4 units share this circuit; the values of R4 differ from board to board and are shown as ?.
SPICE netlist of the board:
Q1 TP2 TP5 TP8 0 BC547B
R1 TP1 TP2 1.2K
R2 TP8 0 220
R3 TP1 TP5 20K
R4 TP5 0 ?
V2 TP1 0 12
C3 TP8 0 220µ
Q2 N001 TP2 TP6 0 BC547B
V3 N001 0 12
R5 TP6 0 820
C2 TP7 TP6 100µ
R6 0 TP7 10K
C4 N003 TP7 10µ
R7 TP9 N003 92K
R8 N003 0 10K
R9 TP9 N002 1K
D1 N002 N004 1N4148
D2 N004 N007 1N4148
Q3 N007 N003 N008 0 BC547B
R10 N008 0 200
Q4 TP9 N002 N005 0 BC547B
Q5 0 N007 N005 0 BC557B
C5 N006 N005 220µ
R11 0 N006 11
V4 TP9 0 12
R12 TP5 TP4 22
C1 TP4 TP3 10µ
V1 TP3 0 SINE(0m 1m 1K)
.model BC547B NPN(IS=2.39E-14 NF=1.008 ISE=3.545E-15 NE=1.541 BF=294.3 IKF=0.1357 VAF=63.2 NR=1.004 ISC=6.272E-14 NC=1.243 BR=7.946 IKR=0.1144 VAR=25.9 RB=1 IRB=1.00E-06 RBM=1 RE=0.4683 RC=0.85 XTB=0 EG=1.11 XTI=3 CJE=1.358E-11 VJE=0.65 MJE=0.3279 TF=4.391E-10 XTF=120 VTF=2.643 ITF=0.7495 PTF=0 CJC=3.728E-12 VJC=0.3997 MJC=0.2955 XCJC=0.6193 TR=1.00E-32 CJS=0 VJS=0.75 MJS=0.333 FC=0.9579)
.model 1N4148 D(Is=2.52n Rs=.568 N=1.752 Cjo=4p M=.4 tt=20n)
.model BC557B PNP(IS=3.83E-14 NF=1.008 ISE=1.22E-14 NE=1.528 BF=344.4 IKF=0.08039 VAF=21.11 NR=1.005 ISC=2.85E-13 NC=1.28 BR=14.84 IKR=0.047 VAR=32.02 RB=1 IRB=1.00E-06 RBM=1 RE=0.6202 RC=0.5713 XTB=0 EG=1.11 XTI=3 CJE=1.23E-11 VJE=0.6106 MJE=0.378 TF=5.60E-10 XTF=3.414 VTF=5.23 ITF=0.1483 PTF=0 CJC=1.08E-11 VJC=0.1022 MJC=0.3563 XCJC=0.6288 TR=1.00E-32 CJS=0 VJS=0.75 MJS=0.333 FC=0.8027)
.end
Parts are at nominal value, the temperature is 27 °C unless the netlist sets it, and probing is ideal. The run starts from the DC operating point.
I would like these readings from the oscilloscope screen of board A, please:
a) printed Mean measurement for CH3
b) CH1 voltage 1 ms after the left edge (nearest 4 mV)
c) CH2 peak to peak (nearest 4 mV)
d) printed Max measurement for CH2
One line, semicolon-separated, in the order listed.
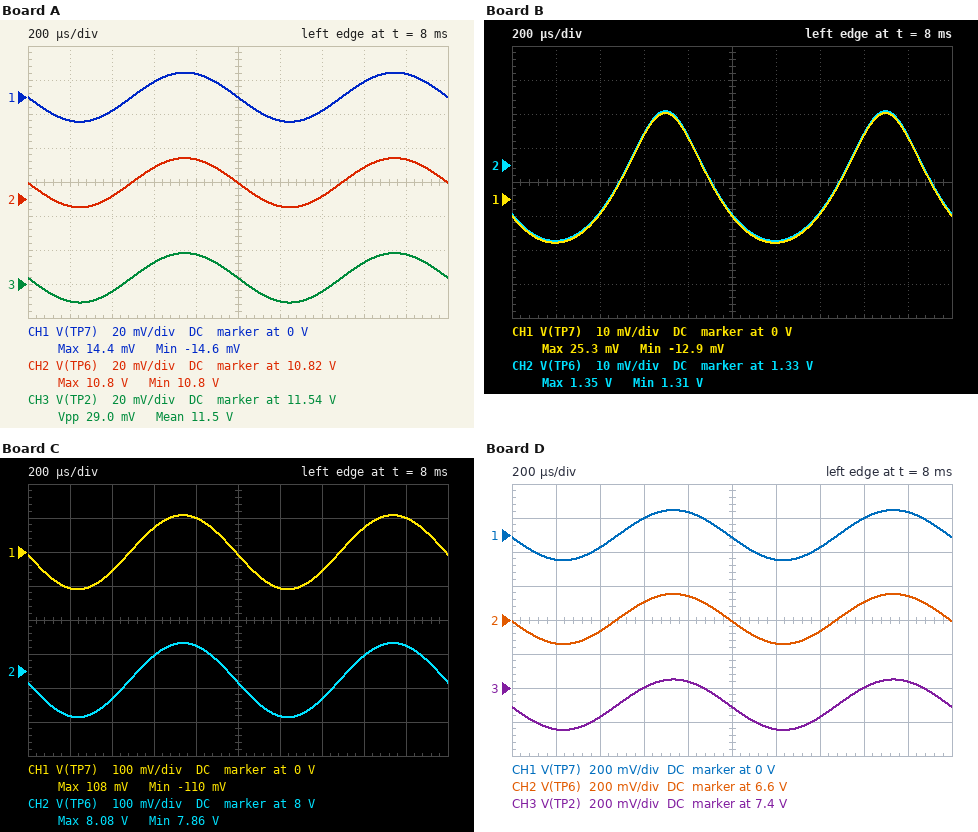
11.5 V; 0 V; 28 mV; 10.8 V
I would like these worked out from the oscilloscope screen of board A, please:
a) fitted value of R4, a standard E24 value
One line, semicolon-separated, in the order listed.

1.2 kΩ
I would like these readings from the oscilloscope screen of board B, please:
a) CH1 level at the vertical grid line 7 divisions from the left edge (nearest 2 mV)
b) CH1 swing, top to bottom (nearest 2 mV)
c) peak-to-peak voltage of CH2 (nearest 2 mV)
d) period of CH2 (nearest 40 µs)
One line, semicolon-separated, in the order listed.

-4 mV; 38 mV; 38 mV; 1.00 ms
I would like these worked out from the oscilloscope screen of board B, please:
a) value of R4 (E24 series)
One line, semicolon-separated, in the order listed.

6.2 kΩ
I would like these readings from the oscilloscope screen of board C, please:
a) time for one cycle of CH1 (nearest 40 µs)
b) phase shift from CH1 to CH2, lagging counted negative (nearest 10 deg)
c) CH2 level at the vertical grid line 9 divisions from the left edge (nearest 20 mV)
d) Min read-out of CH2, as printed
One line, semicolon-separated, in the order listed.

1.00 ms; 0 deg; 8.08 V; 7.86 V
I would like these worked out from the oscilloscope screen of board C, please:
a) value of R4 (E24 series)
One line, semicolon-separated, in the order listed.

2.4 kΩ
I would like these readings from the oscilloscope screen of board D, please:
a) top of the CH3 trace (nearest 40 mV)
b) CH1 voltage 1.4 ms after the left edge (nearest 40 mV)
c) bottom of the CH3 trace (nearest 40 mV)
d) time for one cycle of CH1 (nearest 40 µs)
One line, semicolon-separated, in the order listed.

7.44 V; -80 mV; 7.16 V; 1.00 ms
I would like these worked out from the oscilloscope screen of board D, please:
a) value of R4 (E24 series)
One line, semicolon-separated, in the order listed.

3 kΩ
